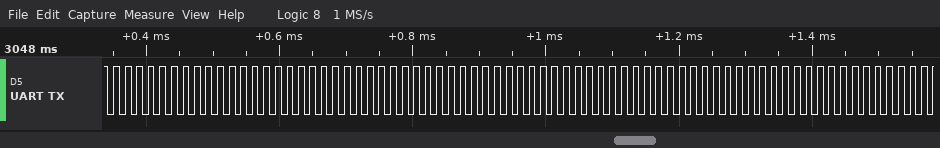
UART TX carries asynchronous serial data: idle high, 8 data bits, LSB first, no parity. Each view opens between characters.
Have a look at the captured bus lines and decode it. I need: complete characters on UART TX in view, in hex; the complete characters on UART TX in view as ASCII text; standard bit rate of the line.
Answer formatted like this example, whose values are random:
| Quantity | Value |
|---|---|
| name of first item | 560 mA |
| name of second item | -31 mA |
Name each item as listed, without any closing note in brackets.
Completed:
| Quantity | Value |
|---|---|
| complete characters on UART TX in view, in hex | 55, 55, 55, 55, 55, 55, 55, 55, 55, 55, 55, 55, 55, 55 |
| the complete characters on UART TX in view as ASCII text | "UUUUUUUUUUUUUU" |
| standard bit rate of the line | 115200 baud |
